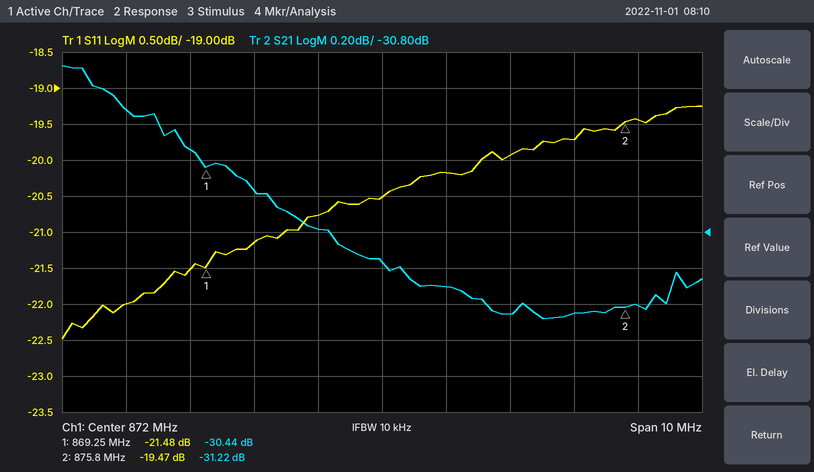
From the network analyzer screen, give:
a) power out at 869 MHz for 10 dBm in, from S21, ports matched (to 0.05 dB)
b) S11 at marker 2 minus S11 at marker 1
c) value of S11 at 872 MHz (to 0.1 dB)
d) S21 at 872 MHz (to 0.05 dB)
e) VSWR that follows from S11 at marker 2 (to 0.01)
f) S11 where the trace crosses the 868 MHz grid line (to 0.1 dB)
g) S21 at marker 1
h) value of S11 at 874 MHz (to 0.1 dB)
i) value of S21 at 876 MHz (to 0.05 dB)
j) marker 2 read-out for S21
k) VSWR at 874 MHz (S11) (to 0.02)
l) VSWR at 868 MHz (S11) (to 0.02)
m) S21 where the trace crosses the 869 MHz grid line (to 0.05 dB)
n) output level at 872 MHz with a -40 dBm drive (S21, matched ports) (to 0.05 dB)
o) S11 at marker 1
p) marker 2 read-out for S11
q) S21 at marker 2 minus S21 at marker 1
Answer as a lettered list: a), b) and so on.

a) -20.35 dBm
b) 2.01 dB
c) -20.5 dB
d) -30.95 dB
e) 1.24
f) -22.0 dB
g) -30.44 dB
h) -19.9 dB
i) -31.20 dB
j) -31.22 dB
k) 1.22
l) 1.18
m) -30.35 dB
n) -70.95 dBm
o) -21.48 dB
p) -19.47 dB
q) -0.78 dB
